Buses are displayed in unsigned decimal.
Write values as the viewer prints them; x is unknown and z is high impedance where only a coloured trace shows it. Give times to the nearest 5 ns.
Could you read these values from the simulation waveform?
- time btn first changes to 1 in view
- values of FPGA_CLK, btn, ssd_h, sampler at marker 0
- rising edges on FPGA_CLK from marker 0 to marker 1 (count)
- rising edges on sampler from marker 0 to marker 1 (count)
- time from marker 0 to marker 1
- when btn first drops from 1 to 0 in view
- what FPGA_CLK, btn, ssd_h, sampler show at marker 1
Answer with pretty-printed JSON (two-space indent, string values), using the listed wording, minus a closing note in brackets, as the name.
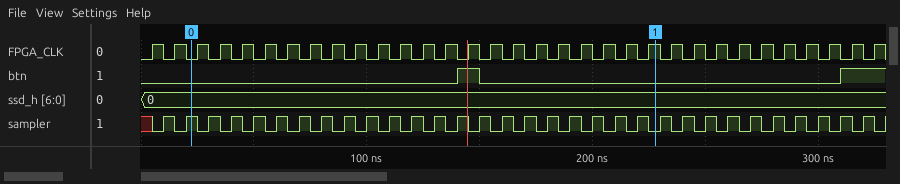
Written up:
{
  "time btn first changes to 1 in view": "140 ns",
  "values of FPGA_CLK, btn, ssd_h, sampler at marker 0": "FPGA_CLK=0, btn=0, ssd_h=0, sampler=1",
  "rising edges on FPGA_CLK from marker 0 to marker 1": "21",
  "rising edges on sampler from marker 0 to marker 1": "20",
  "time from marker 0 to marker 1": "205 ns",
  "when btn first drops from 1 to 0 in view": "150 ns",
  "what FPGA_CLK, btn, ssd_h, sampler show at marker 1": "FPGA_CLK=1, btn=0, ssd_h=0, sampler=0"
}
